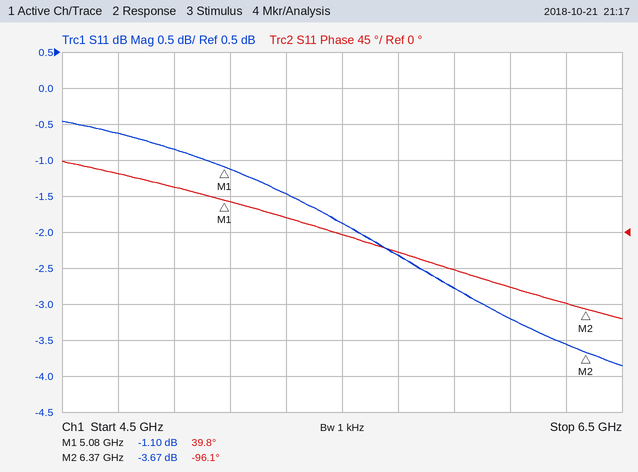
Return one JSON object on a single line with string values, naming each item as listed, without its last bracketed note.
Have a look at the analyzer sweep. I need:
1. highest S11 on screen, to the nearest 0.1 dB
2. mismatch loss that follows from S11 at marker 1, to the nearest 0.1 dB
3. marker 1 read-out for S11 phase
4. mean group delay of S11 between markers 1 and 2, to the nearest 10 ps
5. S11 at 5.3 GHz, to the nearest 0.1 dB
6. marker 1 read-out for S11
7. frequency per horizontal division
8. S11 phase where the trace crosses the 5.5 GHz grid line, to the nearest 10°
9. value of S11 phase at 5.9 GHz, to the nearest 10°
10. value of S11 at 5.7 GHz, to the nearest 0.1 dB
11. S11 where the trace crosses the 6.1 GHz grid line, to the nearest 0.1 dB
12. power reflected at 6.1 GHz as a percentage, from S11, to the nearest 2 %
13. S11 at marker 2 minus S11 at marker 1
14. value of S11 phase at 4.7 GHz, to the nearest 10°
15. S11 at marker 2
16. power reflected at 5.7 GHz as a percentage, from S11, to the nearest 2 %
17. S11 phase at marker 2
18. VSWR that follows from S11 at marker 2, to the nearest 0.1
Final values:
{"highest S11 on screen, to the nearest 0.1 dB": "-0.5 dB", "mismatch loss that follows from S11 at marker 1, to the nearest 0.1 dB": "6.5 dB", "marker 1 read-out for S11 phase": "39.8°", "mean group delay of S11 between markers 1 and 2, to the nearest 10 ps": "290 ps", "S11 at 5.3 GHz, to the nearest 0.1 dB": "-1.5 dB", "marker 1 read-out for S11": "-1.10 dB", "frequency per horizontal division": "200 MHz", "S11 phase where the trace crosses the 5.5 GHz grid line, to the nearest 10°": "0°", "value of S11 phase at 5.9 GHz, to the nearest 10°": "-50°", "value of S11 at 5.7 GHz, to the nearest 0.1 dB": "-2.3 dB", "S11 where the trace crosses the 6.1 GHz grid line, to the nearest 0.1 dB": "-3.2 dB", "power reflected at 6.1 GHz as a percentage, from S11, to the nearest 2 %": "48 %", "S11 at marker 2 minus S11 at marker 1": "-2.57 dB", "value of S11 phase at 4.7 GHz, to the nearest 10°": "70°", "S11 at marker 2": "-3.67 dB", "power reflected at 5.7 GHz as a percentage, from S11, to the nearest 2 %": "58 %", "S11 phase at marker 2": "-96.1°", "VSWR that follows from S11 at marker 2, to the nearest 0.1": "4.8"}
